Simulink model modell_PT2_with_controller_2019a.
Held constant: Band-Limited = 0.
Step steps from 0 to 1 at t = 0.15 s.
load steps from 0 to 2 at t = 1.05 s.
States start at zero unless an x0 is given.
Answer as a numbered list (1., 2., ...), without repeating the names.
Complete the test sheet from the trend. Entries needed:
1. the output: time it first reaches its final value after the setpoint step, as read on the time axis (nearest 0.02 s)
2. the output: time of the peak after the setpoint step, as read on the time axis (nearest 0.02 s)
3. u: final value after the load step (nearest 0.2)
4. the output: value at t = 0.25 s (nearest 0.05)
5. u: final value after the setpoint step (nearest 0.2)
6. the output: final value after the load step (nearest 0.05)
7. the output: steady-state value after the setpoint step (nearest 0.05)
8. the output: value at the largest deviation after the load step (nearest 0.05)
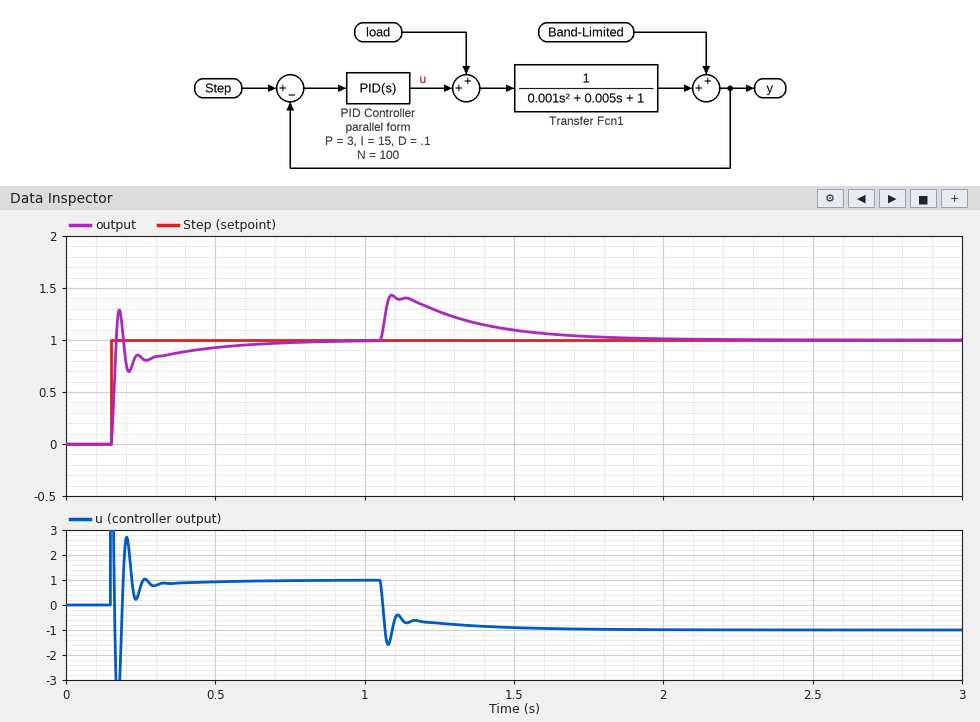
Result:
1. 0.16 s
2. 0.18 s
3. -1.0
4. 0.85
5. 1.0
6. 1.00
7. 1.00
8. 1.45
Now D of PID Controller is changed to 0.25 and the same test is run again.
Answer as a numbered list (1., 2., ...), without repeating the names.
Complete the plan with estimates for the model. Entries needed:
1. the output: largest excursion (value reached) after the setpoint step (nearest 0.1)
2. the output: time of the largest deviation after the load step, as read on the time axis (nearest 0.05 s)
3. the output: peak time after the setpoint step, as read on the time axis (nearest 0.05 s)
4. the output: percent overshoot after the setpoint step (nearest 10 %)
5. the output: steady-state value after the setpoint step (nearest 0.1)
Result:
1. 1.4
2. 1.20 s
3. 0.15 s
4. 40 %
5. 1.0
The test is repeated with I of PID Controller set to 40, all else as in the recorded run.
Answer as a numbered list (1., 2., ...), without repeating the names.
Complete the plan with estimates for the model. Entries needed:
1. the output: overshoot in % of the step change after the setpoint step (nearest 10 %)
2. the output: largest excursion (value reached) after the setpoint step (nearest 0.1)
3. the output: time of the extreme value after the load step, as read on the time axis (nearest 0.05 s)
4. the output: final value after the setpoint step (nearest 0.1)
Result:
1. 30 %
2. 1.3
3. 1.10 s
4. 1.0
